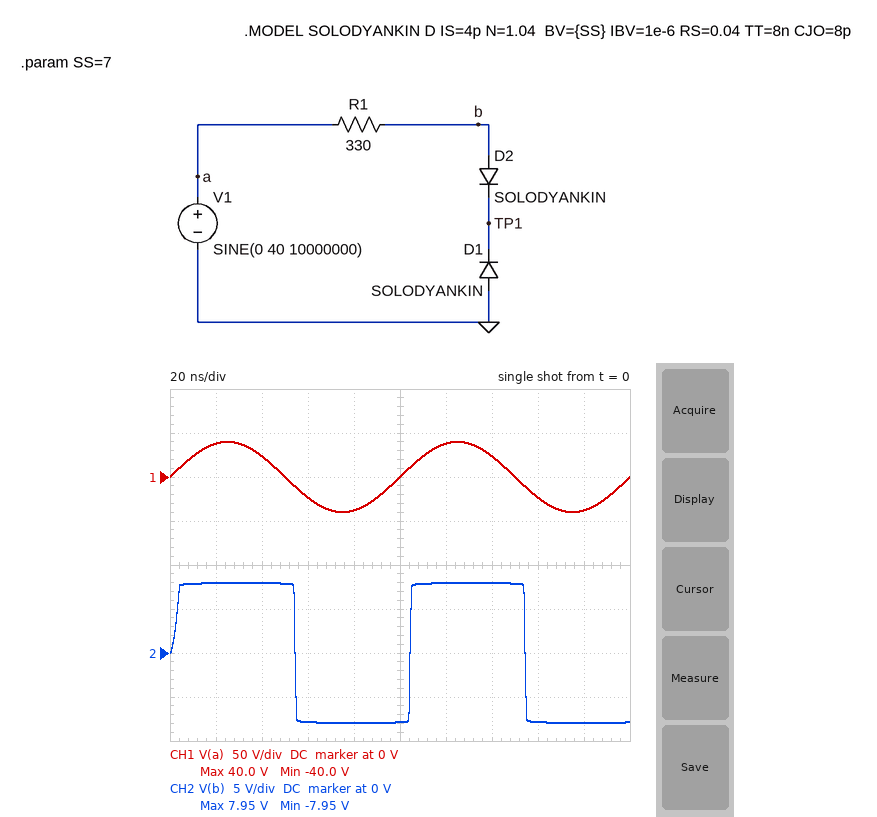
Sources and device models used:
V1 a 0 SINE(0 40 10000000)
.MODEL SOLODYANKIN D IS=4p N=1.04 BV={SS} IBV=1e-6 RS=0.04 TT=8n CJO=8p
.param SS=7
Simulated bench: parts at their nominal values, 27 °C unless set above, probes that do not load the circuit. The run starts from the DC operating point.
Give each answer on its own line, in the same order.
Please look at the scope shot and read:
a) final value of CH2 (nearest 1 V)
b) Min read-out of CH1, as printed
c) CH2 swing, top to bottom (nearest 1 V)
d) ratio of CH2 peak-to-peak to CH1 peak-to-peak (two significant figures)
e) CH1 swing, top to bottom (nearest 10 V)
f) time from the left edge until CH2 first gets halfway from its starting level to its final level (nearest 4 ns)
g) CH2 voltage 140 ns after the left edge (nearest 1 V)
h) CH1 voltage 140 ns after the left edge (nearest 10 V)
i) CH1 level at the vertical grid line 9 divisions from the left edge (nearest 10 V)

-8 V
-40.0 V
16 V
0.20
80 V
56 ns
8 V
20 V
-40 V
